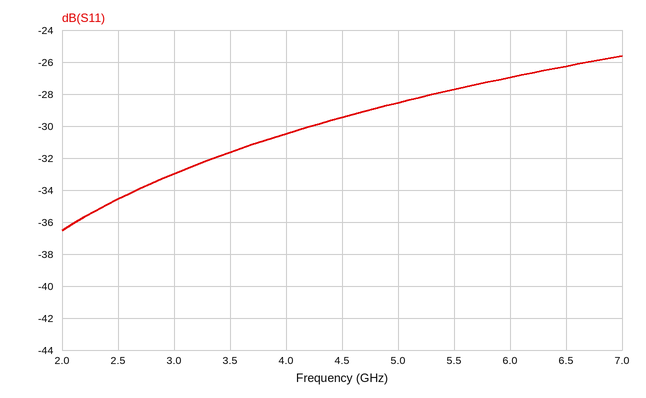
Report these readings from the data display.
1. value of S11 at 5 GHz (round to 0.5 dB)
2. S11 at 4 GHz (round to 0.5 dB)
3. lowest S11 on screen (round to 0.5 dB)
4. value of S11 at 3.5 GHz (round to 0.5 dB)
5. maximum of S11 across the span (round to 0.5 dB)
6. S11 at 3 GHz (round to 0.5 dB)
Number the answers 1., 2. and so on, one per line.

1. -28.5 dB
2. -30.5 dB
3. -36.5 dB
4. -31.5 dB
5. -25.5 dB
6. -33.0 dB
